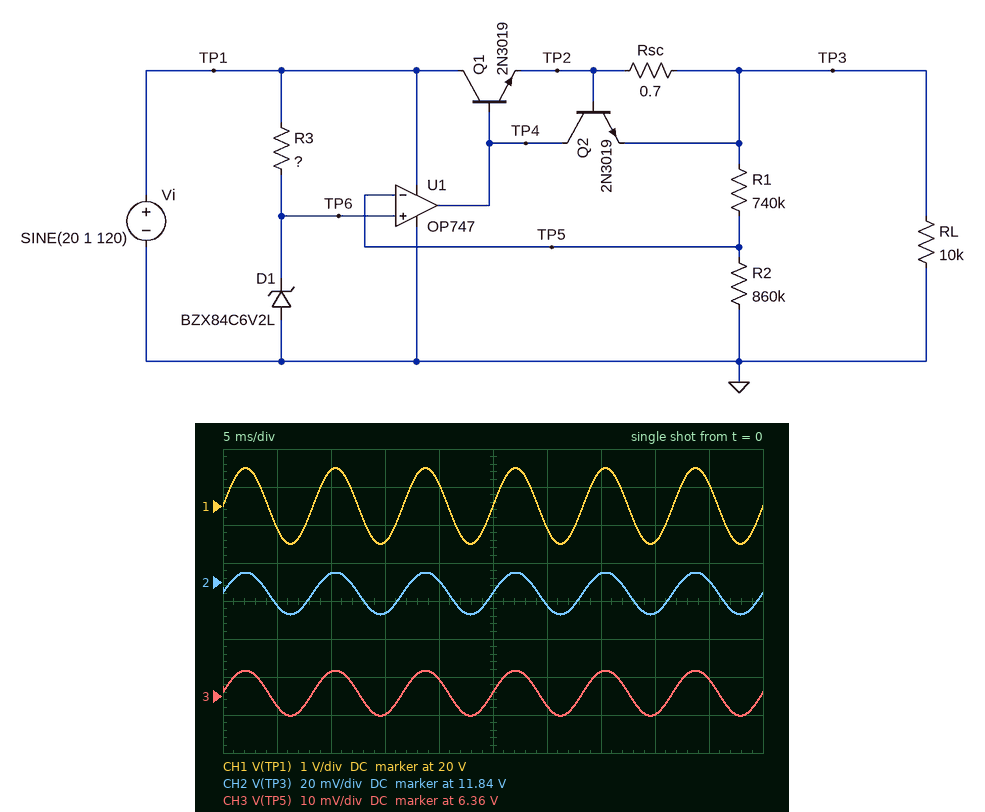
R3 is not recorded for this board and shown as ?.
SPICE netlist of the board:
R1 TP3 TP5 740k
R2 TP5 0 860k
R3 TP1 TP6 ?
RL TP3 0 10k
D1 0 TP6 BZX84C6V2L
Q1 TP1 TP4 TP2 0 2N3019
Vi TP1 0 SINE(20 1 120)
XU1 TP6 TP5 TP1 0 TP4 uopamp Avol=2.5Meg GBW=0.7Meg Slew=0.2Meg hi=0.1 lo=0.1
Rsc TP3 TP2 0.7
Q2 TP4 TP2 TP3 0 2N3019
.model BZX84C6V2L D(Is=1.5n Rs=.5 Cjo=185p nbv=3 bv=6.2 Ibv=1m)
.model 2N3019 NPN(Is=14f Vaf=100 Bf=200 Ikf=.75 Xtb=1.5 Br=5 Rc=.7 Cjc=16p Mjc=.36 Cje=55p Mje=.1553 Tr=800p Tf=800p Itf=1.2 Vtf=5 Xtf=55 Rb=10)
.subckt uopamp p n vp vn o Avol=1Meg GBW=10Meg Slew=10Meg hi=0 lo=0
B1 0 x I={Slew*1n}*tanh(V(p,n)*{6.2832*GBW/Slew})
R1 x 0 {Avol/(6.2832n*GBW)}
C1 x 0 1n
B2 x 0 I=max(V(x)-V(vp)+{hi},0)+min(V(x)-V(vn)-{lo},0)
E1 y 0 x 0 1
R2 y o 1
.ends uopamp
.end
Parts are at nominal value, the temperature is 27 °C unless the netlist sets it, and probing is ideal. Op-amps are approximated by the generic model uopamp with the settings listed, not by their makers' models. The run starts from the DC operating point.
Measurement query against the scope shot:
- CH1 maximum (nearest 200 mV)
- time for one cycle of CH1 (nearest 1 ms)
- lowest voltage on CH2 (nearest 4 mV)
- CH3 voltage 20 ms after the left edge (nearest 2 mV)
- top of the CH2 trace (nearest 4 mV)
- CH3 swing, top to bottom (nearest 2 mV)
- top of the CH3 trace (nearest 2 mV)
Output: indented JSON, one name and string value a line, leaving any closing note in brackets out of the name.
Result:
{
  "CH1 maximum": "21.0 V",
  "time for one cycle of CH1": "8 ms",
  "lowest voltage on CH2": "11.824 V",
  "CH3 voltage 20 ms after the left edge": "6.364 V",
  "top of the CH2 trace": "11.844 V",
  "CH3 swing, top to bottom": "12 mV",
  "top of the CH3 trace": "6.366 V"
}
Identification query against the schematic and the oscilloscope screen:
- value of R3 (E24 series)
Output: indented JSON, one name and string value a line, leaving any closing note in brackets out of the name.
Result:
{
  "value of R3": "1.8 kΩ"
}
